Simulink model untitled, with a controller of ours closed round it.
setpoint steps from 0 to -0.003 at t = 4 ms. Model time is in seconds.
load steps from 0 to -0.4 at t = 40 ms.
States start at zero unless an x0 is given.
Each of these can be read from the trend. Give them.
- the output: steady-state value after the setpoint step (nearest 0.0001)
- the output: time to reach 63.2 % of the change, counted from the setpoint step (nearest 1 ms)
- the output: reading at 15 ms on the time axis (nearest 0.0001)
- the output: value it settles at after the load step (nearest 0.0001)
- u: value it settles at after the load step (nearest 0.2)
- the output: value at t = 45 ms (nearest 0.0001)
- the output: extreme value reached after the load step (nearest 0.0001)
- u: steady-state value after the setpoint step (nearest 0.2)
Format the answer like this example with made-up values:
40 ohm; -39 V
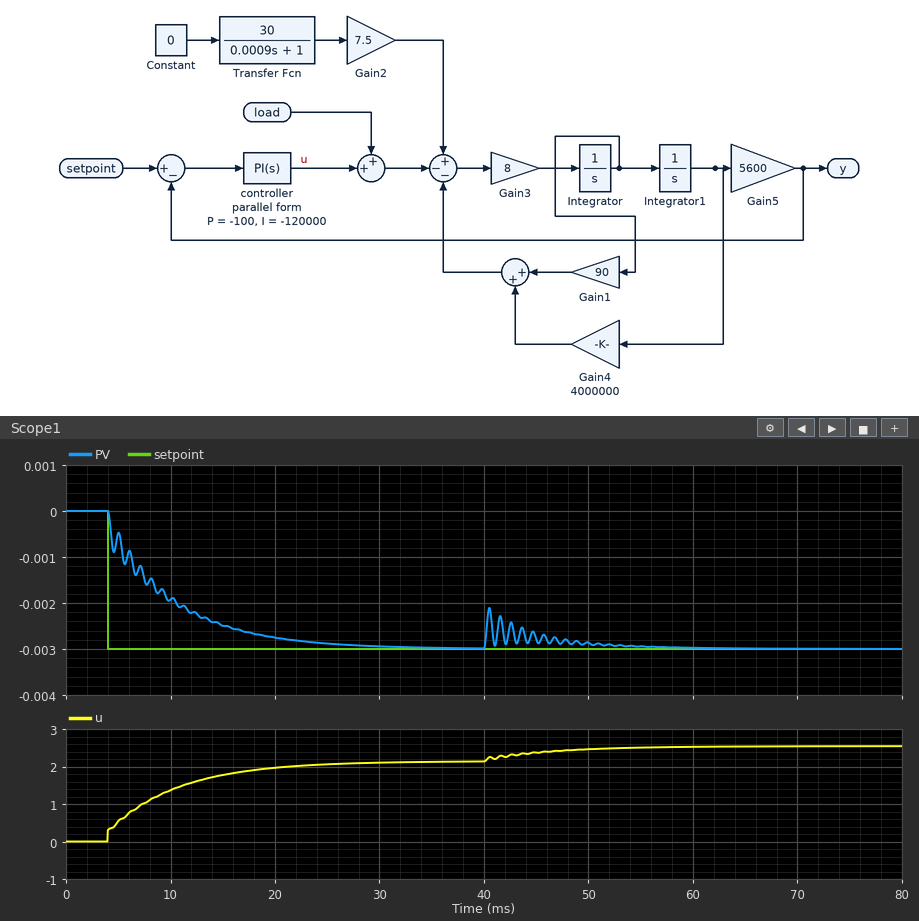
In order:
-0.0030; 6 ms; -0.0025; -0.0030; 2.6; -0.0028; -0.0021; 2.2
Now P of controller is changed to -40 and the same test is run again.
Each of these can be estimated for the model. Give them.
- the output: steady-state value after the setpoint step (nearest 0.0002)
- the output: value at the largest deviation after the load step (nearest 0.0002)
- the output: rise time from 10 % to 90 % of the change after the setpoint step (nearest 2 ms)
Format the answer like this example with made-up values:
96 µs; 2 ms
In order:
-0.0030; -0.0020; 14 ms
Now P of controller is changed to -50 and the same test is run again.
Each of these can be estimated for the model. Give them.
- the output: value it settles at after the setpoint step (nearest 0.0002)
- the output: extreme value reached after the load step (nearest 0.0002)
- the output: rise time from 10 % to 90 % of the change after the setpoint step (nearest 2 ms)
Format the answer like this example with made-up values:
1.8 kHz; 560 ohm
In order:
-0.0030; -0.0020; 14 ms
